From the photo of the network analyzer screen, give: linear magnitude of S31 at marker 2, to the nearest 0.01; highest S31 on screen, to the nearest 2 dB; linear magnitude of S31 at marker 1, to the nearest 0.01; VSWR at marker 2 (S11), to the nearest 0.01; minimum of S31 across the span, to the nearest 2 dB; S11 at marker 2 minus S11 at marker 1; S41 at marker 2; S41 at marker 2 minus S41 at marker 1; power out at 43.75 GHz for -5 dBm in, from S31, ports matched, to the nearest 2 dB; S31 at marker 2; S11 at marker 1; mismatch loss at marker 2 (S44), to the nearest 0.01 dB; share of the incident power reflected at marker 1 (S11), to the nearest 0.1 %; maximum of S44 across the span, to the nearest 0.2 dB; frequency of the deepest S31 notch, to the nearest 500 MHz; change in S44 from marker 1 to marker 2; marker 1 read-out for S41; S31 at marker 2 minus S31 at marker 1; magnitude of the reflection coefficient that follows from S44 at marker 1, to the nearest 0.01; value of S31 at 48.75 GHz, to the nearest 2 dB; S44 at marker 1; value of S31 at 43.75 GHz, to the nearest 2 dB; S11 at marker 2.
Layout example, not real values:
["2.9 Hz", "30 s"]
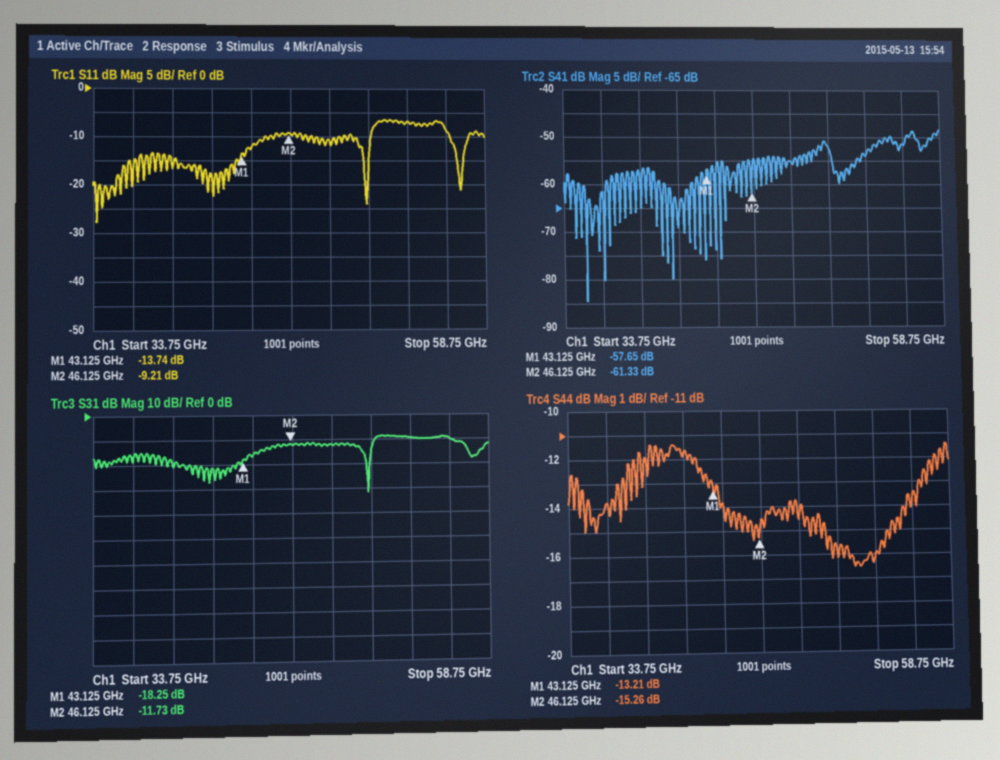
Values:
["0.26", "-8 dB", "0.12", "2.06", "-32 dB", "4.53 dB", "-61.33 dB", "-3.68 dB", "-22 dBm", "-11.73 dB", "-13.74 dB", "0.13 dB", "4.2 %", "-11.4 dB", "51.0 GHz", "-2.05 dB", "-57.65 dB", "6.52 dB", "0.22", "-12 dB", "-13.21 dB", "-16 dB", "-9.21 dB"]
